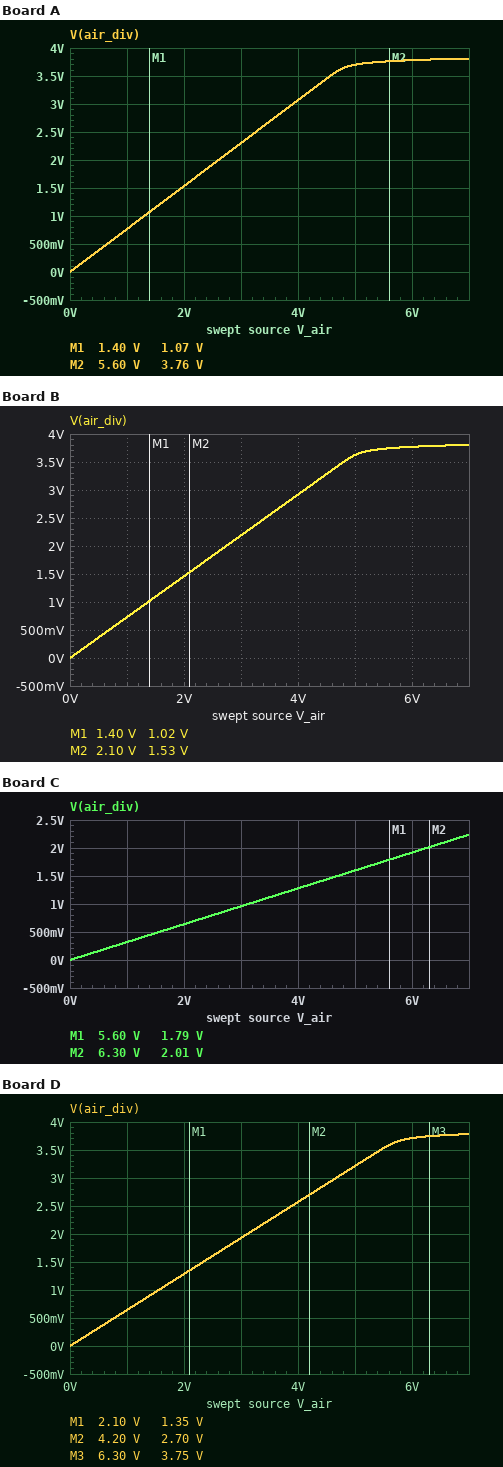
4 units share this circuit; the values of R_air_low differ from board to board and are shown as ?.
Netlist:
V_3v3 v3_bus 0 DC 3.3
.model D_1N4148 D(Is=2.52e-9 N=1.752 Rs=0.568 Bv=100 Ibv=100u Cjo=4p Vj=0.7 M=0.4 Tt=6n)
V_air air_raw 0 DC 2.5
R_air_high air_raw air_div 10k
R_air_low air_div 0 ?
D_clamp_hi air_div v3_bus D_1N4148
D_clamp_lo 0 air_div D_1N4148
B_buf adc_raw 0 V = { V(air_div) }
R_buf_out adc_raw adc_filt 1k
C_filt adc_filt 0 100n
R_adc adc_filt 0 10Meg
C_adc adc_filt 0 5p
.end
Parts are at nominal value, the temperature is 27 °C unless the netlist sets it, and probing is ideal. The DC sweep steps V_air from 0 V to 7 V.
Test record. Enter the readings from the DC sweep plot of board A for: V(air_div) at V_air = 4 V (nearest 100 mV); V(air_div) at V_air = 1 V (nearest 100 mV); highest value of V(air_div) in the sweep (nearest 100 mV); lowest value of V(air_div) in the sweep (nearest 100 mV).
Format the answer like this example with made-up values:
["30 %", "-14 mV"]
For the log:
["3.1 V", "800 mV", "3.8 V", "0 V"]
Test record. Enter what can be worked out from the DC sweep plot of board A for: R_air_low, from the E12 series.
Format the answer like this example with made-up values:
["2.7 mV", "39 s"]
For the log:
["33 kΩ"]
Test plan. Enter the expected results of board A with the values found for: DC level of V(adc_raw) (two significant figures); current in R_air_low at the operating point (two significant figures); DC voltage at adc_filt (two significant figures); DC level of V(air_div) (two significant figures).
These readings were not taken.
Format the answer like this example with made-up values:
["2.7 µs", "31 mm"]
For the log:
["1.9 V", "58 µA", "1.9 V", "1.9 V"]
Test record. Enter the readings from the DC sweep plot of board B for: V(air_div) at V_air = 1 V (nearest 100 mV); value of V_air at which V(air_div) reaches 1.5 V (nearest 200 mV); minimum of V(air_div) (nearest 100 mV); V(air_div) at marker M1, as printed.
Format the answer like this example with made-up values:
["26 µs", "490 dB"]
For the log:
["700 mV", "2.0 V", "0 V", "1.02 V"]
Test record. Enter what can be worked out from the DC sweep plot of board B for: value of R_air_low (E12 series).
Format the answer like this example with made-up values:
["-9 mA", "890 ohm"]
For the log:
["27 kΩ"]
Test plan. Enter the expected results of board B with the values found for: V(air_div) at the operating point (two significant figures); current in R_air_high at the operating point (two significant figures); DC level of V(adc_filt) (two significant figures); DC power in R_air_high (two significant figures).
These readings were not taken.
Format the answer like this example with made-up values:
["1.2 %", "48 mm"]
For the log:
["1.8 V", "68 µA", "1.8 V", "46 µW"]
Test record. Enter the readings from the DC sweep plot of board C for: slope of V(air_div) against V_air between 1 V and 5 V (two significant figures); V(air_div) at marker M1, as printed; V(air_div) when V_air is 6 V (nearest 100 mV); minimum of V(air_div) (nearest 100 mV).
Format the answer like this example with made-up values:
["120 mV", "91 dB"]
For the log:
["0.32 V/V", "1.79 V", "1.9 V", "0 V"]
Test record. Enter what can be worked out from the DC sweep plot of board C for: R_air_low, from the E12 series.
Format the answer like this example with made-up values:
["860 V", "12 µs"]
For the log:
["4.7 kΩ"]
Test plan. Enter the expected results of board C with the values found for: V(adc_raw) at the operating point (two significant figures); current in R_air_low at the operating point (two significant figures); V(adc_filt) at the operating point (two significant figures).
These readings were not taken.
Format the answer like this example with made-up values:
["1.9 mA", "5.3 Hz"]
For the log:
["800 mV", "170 µA", "800 mV"]
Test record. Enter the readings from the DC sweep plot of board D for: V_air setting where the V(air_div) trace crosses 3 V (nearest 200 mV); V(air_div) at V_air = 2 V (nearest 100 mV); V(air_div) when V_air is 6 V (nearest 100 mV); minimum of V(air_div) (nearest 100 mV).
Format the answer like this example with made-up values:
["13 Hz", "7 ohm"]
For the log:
["4.6 V", "1.3 V", "3.7 V", "0 V"]
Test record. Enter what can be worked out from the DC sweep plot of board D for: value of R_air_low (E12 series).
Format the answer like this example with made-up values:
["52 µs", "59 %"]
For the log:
["18 kΩ"]
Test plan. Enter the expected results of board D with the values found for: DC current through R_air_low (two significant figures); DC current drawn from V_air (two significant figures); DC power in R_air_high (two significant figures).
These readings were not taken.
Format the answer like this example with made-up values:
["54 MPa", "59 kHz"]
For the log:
["89 µA", "89 µA", "80 µW"]
